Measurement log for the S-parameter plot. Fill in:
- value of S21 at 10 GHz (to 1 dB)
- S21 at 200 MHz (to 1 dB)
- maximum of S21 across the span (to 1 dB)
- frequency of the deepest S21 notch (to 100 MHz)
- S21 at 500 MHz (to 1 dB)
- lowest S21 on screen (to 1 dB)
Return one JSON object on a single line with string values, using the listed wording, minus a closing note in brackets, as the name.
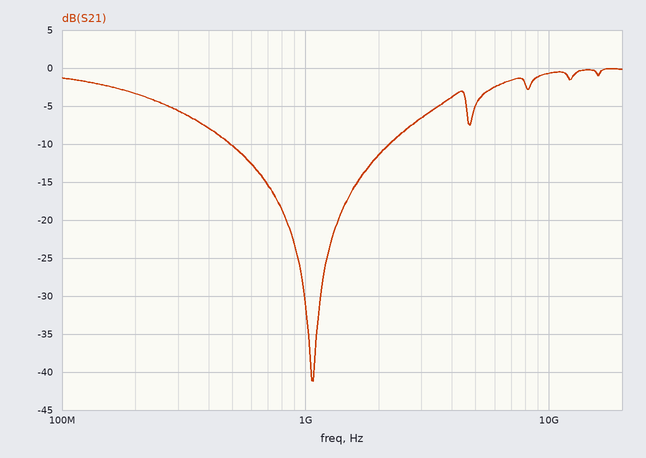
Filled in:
{"value of S21 at 10 GHz": "-1 dB", "S21 at 200 MHz": "-3 dB", "maximum of S21 across the span": "0 dB", "frequency of the deepest S21 notch": "1.1 GHz", "S21 at 500 MHz": "-10 dB", "lowest S21 on screen": "-41 dB"}
